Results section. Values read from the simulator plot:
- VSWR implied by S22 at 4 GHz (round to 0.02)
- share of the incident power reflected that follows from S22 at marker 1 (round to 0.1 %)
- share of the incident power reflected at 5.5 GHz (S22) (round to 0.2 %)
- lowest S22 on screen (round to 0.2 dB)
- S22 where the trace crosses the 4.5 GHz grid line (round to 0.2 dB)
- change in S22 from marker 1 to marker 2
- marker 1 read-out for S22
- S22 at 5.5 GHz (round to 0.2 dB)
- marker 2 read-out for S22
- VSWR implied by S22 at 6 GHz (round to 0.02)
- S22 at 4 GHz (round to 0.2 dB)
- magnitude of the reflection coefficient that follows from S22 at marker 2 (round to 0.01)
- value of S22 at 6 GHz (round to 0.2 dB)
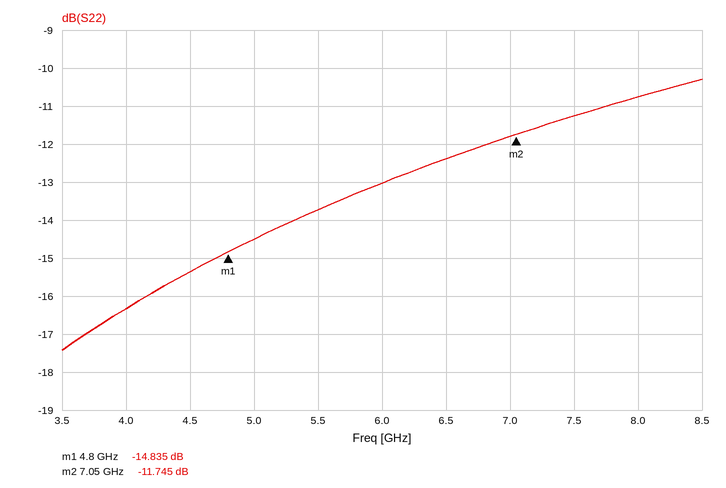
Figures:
1.36
3.3 %
4.2 %
-17.4 dB
-15.4 dB
3.090 dB
-14.835 dB
-13.8 dB
-11.745 dB
1.58
-16.4 dB
0.26
-13.0 dB
